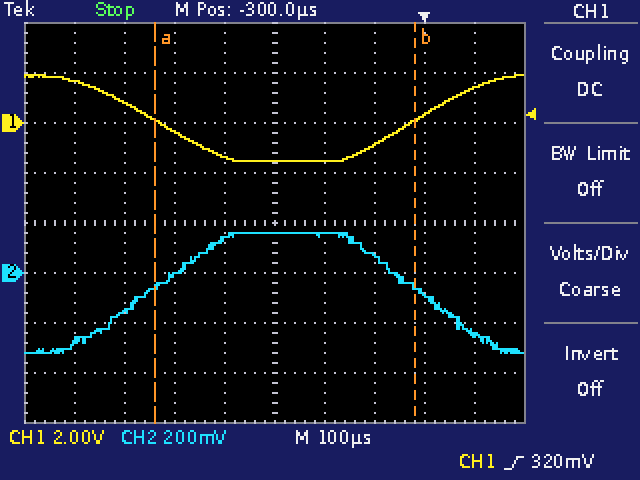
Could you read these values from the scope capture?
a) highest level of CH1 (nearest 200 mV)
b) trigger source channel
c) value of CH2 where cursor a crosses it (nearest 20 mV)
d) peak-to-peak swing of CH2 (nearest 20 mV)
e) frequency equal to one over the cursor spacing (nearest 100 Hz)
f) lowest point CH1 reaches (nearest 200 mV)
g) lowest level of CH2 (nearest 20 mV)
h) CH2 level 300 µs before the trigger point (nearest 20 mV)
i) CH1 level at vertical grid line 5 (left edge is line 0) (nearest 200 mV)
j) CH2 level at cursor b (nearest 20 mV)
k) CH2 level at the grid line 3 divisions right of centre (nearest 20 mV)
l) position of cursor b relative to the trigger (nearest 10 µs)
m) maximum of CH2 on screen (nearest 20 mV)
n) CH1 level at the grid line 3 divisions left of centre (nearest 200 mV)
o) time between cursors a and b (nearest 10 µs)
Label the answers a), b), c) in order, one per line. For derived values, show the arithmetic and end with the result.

a) 2.0 V
b) CH1
c) -60 mV
d) 160 mV − (-320 mV) = 480 mV
e) 1 / 520 µs ≈ 1.9 kHz
f) -1.6 V
g) -320 mV
h) 160 mV
i) -1.6 V
j) -60 mV
k) -80 mV
l) -20 µs
m) 160 mV
n) 800 mV
o) 520 µs
